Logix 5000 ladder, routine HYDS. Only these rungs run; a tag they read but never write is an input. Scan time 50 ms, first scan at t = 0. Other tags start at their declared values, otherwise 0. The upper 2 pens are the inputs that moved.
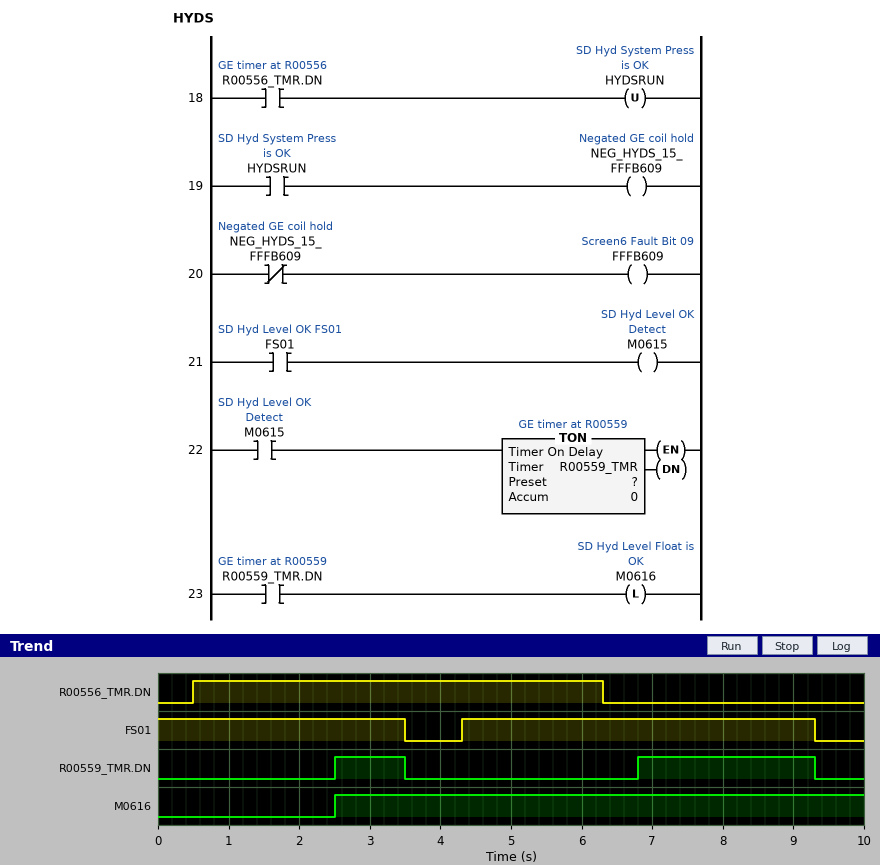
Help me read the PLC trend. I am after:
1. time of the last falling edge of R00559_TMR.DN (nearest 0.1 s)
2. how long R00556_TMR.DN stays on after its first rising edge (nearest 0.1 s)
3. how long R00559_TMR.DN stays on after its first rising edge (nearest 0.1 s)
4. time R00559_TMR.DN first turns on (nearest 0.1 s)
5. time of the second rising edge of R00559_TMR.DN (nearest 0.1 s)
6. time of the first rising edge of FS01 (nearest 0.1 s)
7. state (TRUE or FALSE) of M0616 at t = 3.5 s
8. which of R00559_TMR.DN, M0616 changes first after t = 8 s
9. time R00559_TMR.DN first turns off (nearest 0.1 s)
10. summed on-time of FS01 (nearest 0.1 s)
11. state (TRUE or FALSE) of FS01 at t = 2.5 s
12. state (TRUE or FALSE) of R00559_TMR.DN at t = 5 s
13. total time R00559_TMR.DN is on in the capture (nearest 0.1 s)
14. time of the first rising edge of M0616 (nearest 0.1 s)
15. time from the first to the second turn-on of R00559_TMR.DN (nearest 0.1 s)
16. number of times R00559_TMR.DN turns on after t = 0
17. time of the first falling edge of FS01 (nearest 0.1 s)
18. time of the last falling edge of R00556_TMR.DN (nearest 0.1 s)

9.3 s
5.8 s
1.0 s
2.5 s
6.8 s
4.3 s
TRUE
R00559_TMR.DN
3.5 s
8.5 s
TRUE
FALSE
3.5 s
2.5 s
4.3 s
2
3.5 s
6.3 s
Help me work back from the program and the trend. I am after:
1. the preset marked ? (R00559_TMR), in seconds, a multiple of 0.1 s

2.5 s
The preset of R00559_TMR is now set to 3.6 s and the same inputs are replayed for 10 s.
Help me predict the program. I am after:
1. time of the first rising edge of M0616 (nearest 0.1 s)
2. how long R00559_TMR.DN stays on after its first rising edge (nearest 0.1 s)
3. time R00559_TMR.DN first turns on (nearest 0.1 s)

7.9 s
1.4 s
7.9 s
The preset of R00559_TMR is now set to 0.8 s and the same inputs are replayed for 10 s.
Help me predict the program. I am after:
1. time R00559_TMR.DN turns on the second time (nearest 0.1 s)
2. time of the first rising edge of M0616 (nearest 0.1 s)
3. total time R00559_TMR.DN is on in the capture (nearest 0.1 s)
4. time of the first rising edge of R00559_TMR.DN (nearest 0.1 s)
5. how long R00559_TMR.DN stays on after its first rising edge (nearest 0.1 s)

5.1 s
0.8 s
6.9 s
0.8 s
2.7 s
